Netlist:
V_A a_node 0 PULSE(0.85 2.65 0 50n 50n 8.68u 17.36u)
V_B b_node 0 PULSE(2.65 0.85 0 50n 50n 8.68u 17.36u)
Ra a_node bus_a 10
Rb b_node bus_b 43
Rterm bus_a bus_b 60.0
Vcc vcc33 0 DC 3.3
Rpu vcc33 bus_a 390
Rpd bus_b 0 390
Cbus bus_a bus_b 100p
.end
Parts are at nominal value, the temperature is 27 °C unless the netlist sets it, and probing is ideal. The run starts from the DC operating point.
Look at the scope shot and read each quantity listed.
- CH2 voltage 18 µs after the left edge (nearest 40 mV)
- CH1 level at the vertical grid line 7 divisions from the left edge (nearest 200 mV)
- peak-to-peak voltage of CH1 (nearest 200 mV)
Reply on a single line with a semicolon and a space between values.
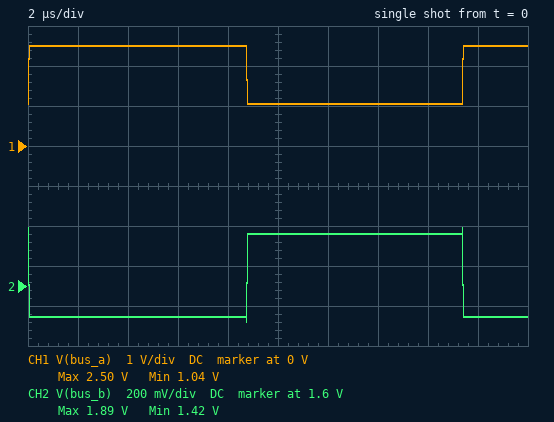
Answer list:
1.44 V; 1.0 V; 1.4 V
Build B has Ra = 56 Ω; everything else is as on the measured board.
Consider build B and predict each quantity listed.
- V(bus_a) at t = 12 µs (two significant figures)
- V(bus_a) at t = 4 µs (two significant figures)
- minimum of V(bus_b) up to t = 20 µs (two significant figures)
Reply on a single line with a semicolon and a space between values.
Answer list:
1.6 V; 2.1 V; 1.3 V
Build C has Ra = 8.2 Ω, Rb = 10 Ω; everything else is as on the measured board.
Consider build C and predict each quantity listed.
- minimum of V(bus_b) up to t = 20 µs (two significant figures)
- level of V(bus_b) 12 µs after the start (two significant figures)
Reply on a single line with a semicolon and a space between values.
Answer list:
1.1 V; 2.4 V
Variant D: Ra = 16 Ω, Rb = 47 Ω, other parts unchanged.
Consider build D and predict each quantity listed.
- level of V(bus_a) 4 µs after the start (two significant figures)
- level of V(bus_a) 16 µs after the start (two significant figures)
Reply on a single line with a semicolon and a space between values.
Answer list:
2.4 V; 1.1 V
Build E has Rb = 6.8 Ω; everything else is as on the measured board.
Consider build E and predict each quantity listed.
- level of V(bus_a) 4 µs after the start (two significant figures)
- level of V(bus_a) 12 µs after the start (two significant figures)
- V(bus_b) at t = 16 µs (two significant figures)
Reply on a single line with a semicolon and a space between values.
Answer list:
2.4 V; 1.1 V; 2.5 V
